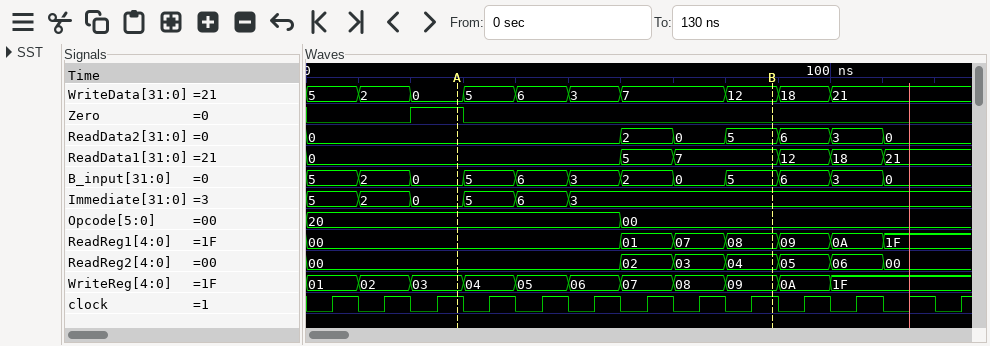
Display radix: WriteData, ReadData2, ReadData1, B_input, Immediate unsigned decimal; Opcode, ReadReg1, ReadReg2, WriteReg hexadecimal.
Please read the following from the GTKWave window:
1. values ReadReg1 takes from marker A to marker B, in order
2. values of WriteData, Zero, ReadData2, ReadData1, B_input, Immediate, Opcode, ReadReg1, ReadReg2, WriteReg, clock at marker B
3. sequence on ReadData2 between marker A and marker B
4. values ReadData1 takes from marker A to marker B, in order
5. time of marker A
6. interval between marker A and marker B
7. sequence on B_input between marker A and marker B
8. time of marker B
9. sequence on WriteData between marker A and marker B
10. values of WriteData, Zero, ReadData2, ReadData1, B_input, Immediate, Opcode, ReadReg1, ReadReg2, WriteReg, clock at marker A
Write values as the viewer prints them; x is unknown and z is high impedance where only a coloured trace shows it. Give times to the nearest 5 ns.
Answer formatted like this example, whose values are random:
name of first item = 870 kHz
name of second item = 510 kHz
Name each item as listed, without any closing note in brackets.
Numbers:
values ReadReg1 takes from marker A to marker B, in order = 00, 01, 07, 08
values of WriteData, Zero, ReadData2, ReadData1, B_input, Immediate, Opcode, ReadReg1, ReadReg2, WriteReg, clock at marker B = WriteData=12, Zero=0, ReadData2=5, ReadData1=7, B_input=5, Immediate=3, Opcode=00, ReadReg1=08, ReadReg2=04, WriteReg=09, clock=1
sequence on ReadData2 between marker A and marker B = 0, 2, 0, 5
values ReadData1 takes from marker A to marker B, in order = 0, 5, 7
time of marker A = 30 ns
interval between marker A and marker B = 60 ns
sequence on B_input between marker A and marker B = 0, 5, 6, 3, 2, 0, 5
time of marker B = 90 ns
sequence on WriteData between marker A and marker B = 0, 5, 6, 3, 7, 12
values of WriteData, Zero, ReadData2, ReadData1, B_input, Immediate, Opcode, ReadReg1, ReadReg2, WriteReg, clock at marker A = WriteData=0, Zero=1, ReadData2=0, ReadData1=0, B_input=0, Immediate=0, Opcode=20, ReadReg1=00, ReadReg2=00, WriteReg=03, clock=1
